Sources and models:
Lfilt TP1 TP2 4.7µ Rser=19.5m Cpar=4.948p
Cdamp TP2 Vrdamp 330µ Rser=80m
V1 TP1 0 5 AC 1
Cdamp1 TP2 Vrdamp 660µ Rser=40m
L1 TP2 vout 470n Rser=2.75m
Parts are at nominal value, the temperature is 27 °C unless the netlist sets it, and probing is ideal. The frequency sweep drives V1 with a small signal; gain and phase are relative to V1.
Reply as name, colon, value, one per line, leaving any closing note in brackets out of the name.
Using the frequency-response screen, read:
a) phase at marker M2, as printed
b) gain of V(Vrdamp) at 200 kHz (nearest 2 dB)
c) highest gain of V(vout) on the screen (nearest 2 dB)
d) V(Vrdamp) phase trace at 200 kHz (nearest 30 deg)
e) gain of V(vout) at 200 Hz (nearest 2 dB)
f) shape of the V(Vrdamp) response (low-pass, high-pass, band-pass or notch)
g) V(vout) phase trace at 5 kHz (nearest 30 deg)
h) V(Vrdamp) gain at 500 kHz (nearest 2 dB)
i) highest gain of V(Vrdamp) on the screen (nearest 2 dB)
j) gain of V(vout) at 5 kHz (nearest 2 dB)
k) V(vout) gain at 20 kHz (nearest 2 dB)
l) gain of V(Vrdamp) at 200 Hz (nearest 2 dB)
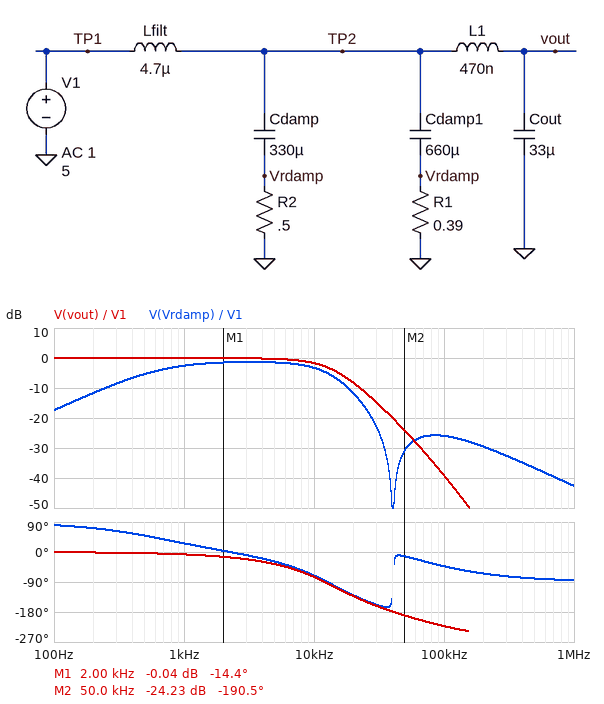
phase at marker M2, as printed: -190.5 deg
gain of V(Vrdamp) at 200 kHz: -30 dB
highest gain of V(vout) on the screen: 0 dB
V(Vrdamp) phase trace at 200 kHz: -60 deg
gain of V(vout) at 200 Hz: 0 dB
shape of the V(Vrdamp) response: band-pass
V(vout) phase trace at 5 kHz: -30 deg
V(Vrdamp) gain at 500 kHz: -36 dB
highest gain of V(Vrdamp) on the screen: -2 dB
gain of V(vout) at 5 kHz: 0 dB
V(vout) gain at 20 kHz: -8 dB
gain of V(Vrdamp) at 200 Hz: -12 dB
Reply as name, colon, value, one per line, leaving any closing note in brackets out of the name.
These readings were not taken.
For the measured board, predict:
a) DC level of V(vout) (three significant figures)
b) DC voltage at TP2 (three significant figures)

DC level of V(vout): 5.00 V
DC voltage at TP2: 5.00 V
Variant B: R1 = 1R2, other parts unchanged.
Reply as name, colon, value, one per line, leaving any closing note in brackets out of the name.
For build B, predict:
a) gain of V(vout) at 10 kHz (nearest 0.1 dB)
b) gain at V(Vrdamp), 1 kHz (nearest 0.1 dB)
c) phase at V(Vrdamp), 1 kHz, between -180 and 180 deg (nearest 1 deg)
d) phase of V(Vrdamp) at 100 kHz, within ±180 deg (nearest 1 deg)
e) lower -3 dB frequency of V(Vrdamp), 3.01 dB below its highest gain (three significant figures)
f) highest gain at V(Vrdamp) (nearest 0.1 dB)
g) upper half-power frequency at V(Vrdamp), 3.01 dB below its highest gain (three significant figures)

gain of V(vout) at 10 kHz: 1.4 dB
gain at V(Vrdamp), 1 kHz: -1.5 dB
phase at V(Vrdamp), 1 kHz, between -180 and 180 deg: 18 deg
phase of V(Vrdamp) at 100 kHz, within ±180 deg: -31 deg
lower -3 dB frequency of V(Vrdamp), 3.01 dB below its highest gain: 565 Hz
highest gain at V(Vrdamp): 0.3 dB
upper half-power frequency at V(Vrdamp), 3.01 dB below its highest gain: 14.3 kHz
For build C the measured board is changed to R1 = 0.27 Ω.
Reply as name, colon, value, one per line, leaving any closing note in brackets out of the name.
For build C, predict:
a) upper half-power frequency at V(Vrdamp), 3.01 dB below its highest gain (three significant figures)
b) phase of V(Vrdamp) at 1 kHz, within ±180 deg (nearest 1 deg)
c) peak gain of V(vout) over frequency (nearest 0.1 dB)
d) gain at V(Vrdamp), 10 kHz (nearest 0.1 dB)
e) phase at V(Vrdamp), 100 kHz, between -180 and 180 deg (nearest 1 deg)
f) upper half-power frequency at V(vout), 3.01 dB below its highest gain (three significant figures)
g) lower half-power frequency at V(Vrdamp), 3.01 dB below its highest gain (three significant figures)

upper half-power frequency at V(Vrdamp), 3.01 dB below its highest gain: 9.61 kHz
phase of V(Vrdamp) at 1 kHz, within ±180 deg: 30 deg
peak gain of V(vout) over frequency: 0.1 dB
gain at V(Vrdamp), 10 kHz: -5.0 dB
phase at V(Vrdamp), 100 kHz, between -180 and 180 deg: -48 deg
upper half-power frequency at V(vout), 3.01 dB below its highest gain: 9.49 kHz
lower half-power frequency at V(Vrdamp), 3.01 dB below its highest gain: 701 Hz
